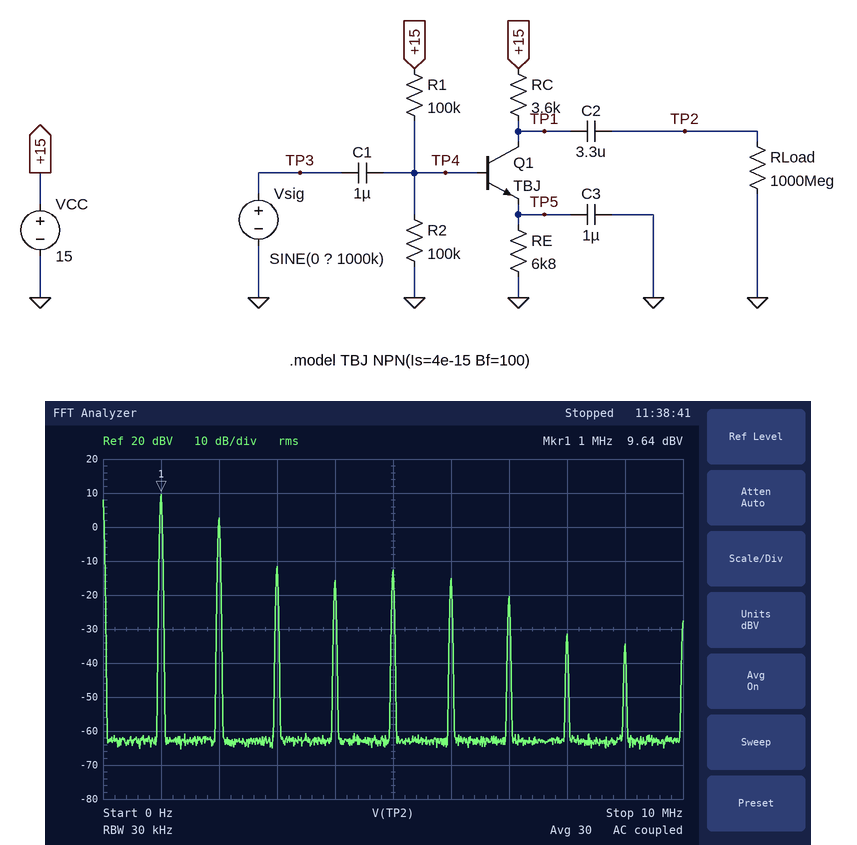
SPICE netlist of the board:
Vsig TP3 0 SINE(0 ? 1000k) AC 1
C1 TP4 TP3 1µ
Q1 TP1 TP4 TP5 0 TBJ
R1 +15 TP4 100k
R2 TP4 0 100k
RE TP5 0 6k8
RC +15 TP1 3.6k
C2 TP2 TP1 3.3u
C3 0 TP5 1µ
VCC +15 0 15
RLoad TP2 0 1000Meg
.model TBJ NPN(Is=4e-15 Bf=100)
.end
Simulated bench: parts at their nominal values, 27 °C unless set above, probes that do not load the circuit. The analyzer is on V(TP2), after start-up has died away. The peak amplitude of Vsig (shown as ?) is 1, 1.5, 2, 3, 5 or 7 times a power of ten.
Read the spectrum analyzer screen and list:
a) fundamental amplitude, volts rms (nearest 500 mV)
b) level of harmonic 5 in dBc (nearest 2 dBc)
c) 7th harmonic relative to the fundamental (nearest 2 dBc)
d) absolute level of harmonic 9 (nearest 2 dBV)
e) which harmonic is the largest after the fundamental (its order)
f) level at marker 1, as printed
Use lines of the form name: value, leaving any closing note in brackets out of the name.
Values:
fundamental amplitude, volts rms: 3.0 V
level of harmonic 5 in dBc: -22 dBc
7th harmonic relative to the fundamental: -30 dBc
absolute level of harmonic 9: -34 dBV
which harmonic is the largest after the fundamental: 2
level at marker 1, as printed: 9.64 dBV
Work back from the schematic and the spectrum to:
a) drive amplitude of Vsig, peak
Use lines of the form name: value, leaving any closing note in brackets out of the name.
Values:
drive amplitude of Vsig, peak: 70 mV
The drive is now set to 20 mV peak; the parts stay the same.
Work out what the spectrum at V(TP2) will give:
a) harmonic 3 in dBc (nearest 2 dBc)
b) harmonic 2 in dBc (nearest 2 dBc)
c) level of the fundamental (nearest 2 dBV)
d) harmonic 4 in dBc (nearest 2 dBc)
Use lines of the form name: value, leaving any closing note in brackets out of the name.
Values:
harmonic 3 in dBc: -32 dBc
harmonic 2 in dBc: -14 dBc
level of the fundamental: 4 dBV
harmonic 4 in dBc: -52 dBc
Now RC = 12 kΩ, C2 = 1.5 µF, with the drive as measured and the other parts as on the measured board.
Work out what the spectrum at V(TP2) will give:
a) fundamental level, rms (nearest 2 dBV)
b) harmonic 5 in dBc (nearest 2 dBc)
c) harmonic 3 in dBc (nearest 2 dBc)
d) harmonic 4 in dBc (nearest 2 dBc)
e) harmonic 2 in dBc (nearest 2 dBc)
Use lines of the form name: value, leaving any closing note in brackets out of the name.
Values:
fundamental level, rms: 12 dBV
harmonic 5 in dBc: -40 dBc
harmonic 3 in dBc: -14 dBc
harmonic 4 in dBc: -18 dBc
harmonic 2 in dBc: -16 dBc
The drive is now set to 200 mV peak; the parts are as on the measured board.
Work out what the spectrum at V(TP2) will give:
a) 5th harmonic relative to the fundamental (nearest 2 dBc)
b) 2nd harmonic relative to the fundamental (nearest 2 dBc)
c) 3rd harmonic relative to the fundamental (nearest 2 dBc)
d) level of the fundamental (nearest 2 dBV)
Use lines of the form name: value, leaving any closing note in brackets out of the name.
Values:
5th harmonic relative to the fundamental: -24 dBc
2nd harmonic relative to the fundamental: -2 dBc
3rd harmonic relative to the fundamental: -8 dBc
level of the fundamental: 8 dBV
